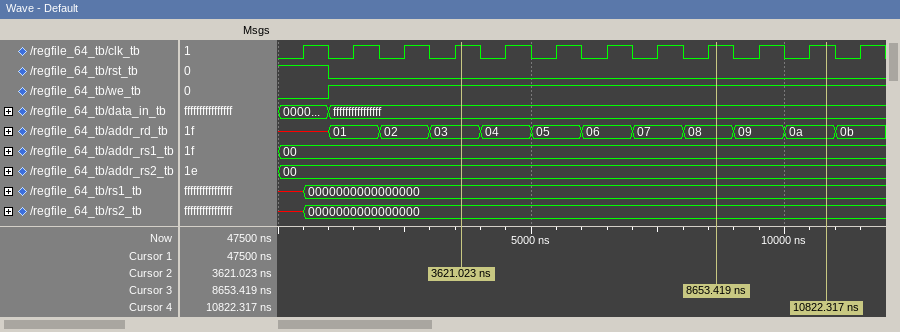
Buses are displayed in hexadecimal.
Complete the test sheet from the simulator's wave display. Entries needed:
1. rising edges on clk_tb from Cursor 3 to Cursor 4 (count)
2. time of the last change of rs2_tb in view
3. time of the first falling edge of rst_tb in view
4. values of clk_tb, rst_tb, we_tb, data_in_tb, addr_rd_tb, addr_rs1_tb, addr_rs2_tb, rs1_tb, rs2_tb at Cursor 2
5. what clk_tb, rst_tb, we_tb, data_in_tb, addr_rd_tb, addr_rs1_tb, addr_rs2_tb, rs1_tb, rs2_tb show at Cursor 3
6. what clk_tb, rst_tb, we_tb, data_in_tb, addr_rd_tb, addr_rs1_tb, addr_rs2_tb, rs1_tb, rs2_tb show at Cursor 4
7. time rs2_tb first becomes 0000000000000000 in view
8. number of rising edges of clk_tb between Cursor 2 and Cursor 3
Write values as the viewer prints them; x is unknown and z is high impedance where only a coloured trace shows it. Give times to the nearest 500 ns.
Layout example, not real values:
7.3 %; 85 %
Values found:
2; 500 ns; 1000 ns; clk_tb=1, rst_tb=0, we_tb=1, data_in_tb=ffffffffffffffff, addr_rd_tb=03, addr_rs1_tb=00, addr_rs2_tb=00, rs1_tb=0000000000000000, rs2_tb=0000000000000000; clk_tb=1, rst_tb=0, we_tb=1, data_in_tb=ffffffffffffffff, addr_rd_tb=08, addr_rs1_tb=00, addr_rs2_tb=00, rs1_tb=0000000000000000, rs2_tb=0000000000000000; clk_tb=1, rst_tb=0, we_tb=1, data_in_tb=ffffffffffffffff, addr_rd_tb=0a, addr_rs1_tb=00, addr_rs2_tb=00, rs1_tb=0000000000000000, rs2_tb=0000000000000000; 500 ns; 5
